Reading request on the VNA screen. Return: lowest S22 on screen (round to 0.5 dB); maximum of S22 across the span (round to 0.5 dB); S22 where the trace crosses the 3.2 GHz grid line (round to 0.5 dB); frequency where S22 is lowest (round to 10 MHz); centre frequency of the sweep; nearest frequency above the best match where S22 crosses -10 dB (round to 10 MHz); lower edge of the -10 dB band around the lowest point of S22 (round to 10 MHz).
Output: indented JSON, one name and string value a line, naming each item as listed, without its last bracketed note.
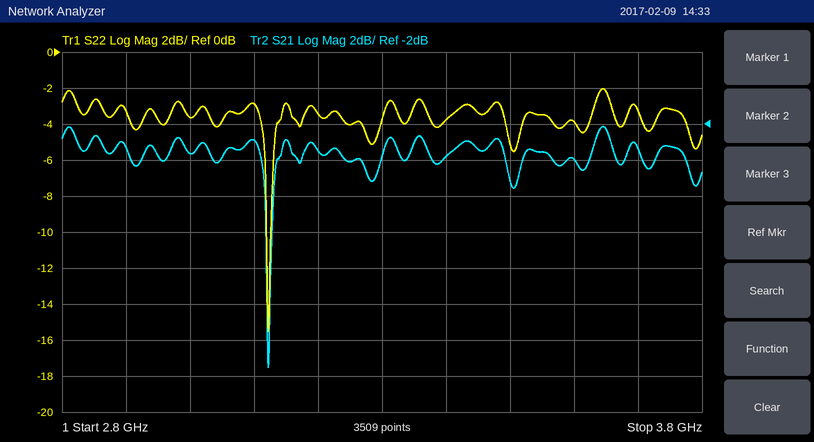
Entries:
{
  "lowest S22 on screen": "-15.5 dB",
  "maximum of S22 across the span": "-2.0 dB",
  "S22 where the trace crosses the 3.2 GHz grid line": "-3.5 dB",
  "frequency where S22 is lowest": "3.12 GHz",
  "centre frequency of the sweep": "3.3 GHz",
  "nearest frequency above the best match where S22 crosses -10 dB": "3.13 GHz",
  "lower edge of the -10 dB band around the lowest point of S22": "3.12 GHz"
}
